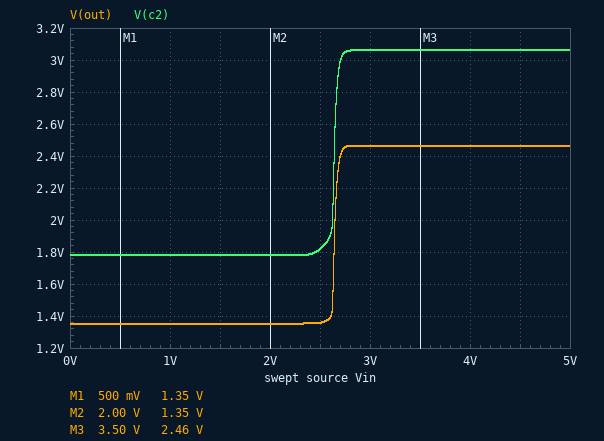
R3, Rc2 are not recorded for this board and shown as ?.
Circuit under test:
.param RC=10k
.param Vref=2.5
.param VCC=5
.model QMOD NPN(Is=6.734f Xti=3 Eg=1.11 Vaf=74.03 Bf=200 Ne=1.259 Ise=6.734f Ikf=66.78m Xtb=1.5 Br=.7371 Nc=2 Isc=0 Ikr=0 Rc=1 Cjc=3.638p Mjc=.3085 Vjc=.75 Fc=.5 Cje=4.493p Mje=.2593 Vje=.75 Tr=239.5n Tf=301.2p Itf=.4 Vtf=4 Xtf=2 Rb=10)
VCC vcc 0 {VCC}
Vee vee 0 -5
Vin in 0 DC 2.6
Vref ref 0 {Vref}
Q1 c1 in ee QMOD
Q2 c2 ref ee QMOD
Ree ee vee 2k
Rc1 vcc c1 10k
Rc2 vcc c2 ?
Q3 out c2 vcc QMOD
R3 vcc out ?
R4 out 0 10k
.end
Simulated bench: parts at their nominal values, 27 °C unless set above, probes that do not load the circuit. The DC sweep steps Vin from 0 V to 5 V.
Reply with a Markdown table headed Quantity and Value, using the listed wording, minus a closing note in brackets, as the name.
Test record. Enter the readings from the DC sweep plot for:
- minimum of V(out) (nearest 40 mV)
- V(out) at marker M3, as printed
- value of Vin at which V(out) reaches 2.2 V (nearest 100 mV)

| Quantity | Value |
|---|---|
| minimum of V(out) | 1.36 V |
| V(out) at marker M3, as printed | 2.46 V |
| value of Vin at which V(out) reaches 2.2 V | 2.7 V |
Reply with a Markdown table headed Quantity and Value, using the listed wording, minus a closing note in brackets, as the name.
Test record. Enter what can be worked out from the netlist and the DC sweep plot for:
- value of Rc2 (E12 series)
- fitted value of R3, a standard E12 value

| Quantity | Value |
|---|---|
| value of Rc2 | 22 kΩ |
| fitted value of R3, a standard E12 value | 27 kΩ |
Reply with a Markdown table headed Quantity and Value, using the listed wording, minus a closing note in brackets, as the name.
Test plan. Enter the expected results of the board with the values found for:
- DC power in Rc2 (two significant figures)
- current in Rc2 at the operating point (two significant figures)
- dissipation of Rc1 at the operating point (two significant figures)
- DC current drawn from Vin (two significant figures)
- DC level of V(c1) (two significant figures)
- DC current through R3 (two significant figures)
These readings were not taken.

| Quantity | Value |
|---|---|
| DC power in Rc2 | 440 µW |
| current in Rc2 at the operating point | 140 µA |
| dissipation of Rc1 at the operating point | 970 µW |
| DC current drawn from Vin | 2.9 mA |
| DC level of V(c1) | 1.9 V |
| DC current through R3 | 130 µA |
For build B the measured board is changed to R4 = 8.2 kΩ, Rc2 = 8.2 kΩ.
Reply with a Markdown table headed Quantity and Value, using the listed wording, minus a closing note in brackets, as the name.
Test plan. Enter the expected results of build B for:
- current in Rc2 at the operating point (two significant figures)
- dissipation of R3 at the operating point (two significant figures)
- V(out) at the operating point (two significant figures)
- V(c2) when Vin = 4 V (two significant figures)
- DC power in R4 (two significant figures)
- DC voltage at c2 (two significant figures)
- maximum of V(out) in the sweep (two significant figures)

| Quantity | Value |
|---|---|
| current in Rc2 at the operating point | 360 µA |
| dissipation of R3 at the operating point | 450 µW |
| V(out) at the operating point | 1.5 V |
| V(c2) when Vin = 4 V | 3.6 V |
| DC power in R4 | 280 µW |
| DC voltage at c2 | 2.1 V |
| maximum of V(out) in the sweep | 3.0 V |
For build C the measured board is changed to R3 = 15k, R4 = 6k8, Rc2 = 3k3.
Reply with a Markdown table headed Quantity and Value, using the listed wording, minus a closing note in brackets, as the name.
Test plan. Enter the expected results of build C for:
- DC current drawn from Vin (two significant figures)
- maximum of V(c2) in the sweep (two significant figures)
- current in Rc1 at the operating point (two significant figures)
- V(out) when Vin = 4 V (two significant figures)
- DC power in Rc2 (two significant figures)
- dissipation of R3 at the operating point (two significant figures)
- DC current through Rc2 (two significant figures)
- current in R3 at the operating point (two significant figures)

| Quantity | Value |
|---|---|
| DC current drawn from Vin | 2.8 mA |
| maximum of V(c2) in the sweep | 4.2 V |
| current in Rc1 at the operating point | 310 µA |
| V(out) when Vin = 4 V | 3.6 V |
| DC power in Rc2 | 770 µW |
| dissipation of R3 at the operating point | 320 µW |
| DC current through Rc2 | 480 µA |
| current in R3 at the operating point | 150 µA |
